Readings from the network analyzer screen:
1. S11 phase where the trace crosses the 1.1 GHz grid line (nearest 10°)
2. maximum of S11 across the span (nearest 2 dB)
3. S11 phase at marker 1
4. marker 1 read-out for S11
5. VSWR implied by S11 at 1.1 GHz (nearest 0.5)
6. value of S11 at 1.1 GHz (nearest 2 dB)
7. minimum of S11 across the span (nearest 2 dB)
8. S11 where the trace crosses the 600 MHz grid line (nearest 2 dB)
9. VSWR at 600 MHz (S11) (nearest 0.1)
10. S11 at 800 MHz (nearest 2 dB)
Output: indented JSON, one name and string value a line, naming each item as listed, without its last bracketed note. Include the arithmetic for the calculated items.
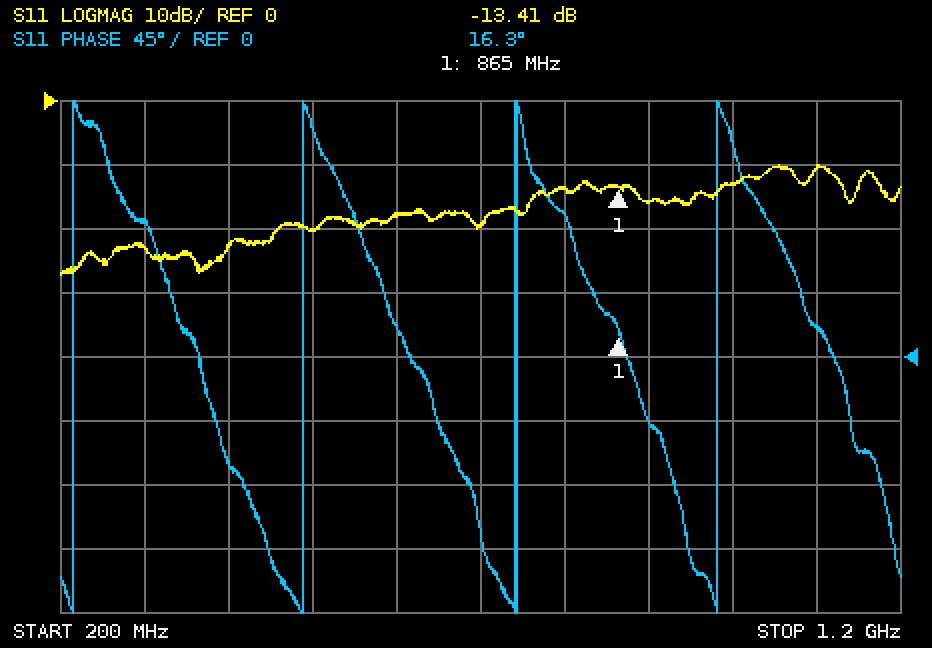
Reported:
{
  "S11 phase where the trace crosses the 1.1 GHz grid line": "20°",
  "maximum of S11 across the span": "-10 dB",
  "S11 phase at marker 1": "16.3°",
  "marker 1 read-out for S11": "-13.41 dB",
  "VSWR implied by S11 at 1.1 GHz": "|Γ| = 10^(-10/20) = 0.3162; VSWR = (1 + 0.3162)/(1 − 0.3162) ≈ 1.92, so 2.0 to the nearest 0.5",
  "value of S11 at 1.1 GHz": "-10 dB",
  "minimum of S11 across the span": "-28 dB",
  "S11 where the trace crosses the 600 MHz grid line": "-18 dB",
  "VSWR at 600 MHz (S11)": "|Γ| = 10^(-18/20) = 0.1259; VSWR = (1 + 0.1259)/(1 − 0.1259) ≈ 1.3",
  "S11 at 800 MHz": "-14 dB"
}
